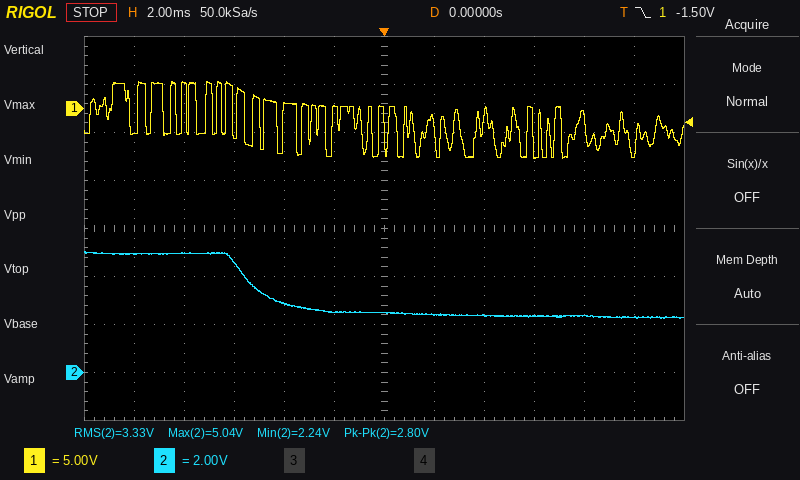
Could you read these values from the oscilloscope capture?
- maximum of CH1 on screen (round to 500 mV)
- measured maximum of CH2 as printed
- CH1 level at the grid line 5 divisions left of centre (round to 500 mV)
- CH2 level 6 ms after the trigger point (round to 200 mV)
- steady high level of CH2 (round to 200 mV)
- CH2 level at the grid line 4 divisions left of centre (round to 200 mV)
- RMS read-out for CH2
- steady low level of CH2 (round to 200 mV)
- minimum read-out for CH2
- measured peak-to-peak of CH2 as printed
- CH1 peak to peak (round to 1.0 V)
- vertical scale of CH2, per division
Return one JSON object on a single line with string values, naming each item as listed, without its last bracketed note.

{"maximum of CH1 on screen": "3.0 V", "measured maximum of CH2 as printed": "5.04 V", "CH1 level at the grid line 5 divisions left of centre": "-2.5 V", "CH2 level 6 ms after the trigger point": "2.4 V", "steady high level of CH2": "5.0 V", "CH2 level at the grid line 4 divisions left of centre": "5.0 V", "RMS read-out for CH2": "3.33 V", "steady low level of CH2": "2.4 V", "minimum read-out for CH2": "2.24 V", "measured peak-to-peak of CH2 as printed": "2.80 V", "CH1 peak to peak": "8.0 V", "vertical scale of CH2, per division": "2 V"}
